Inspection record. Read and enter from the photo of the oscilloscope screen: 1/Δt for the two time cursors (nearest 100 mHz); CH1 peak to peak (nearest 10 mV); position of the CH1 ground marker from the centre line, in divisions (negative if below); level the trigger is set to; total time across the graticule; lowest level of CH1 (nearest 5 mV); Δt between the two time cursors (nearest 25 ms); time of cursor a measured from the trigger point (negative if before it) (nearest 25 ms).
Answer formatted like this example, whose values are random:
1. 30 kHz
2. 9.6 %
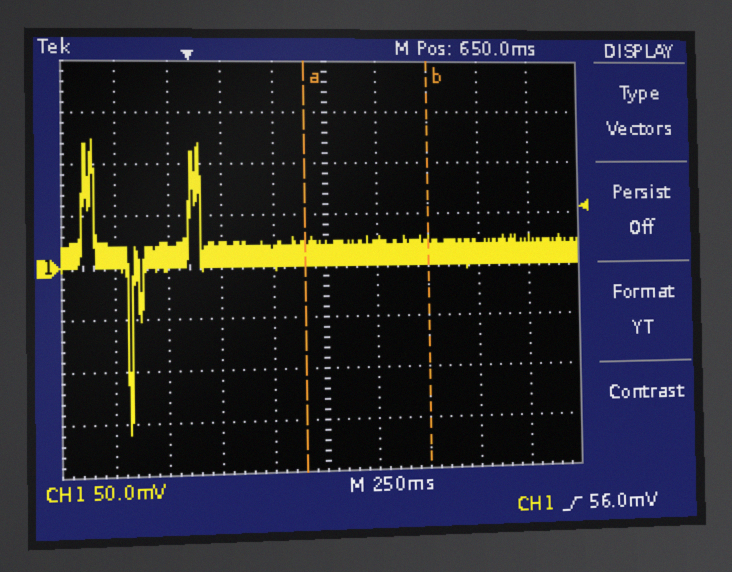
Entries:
1. 1.7 Hz
2. 280 mV
3. 0.0 div
4. 56.0 mV
5. 2.5 s
6. -160 mV
7. 600 ms
8. +550 ms
